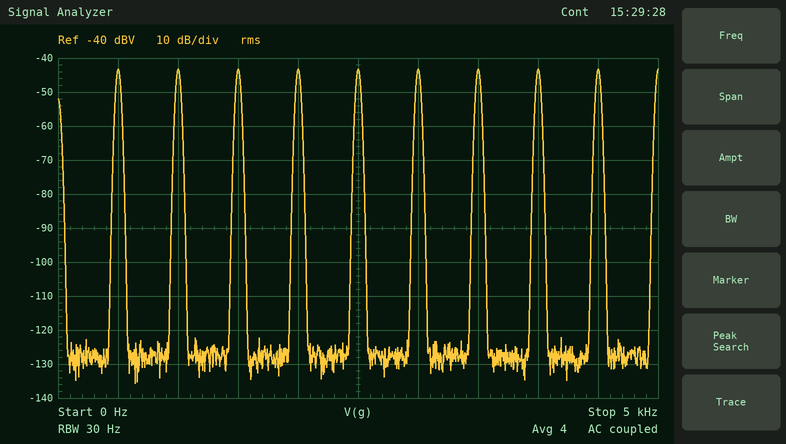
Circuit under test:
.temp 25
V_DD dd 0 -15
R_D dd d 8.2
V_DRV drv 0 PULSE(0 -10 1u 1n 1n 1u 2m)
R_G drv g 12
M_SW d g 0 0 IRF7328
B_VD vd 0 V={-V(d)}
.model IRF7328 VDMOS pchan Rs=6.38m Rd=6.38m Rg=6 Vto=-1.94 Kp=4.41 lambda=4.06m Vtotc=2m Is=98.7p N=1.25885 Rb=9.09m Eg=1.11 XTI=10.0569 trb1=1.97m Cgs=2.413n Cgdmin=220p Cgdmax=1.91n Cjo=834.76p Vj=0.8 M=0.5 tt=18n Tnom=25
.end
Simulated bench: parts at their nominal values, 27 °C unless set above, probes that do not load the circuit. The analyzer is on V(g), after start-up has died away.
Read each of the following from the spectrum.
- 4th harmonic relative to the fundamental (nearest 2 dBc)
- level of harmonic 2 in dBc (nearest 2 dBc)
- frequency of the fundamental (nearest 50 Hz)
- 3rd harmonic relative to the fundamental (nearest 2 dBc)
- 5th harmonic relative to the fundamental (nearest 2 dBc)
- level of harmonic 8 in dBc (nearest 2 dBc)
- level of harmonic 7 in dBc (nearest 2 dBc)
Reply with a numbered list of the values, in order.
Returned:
1. 0 dBc
2. 0 dBc
3. 500 Hz
4. 0 dBc
5. 0 dBc
6. 0 dBc
7. 0 dBc
